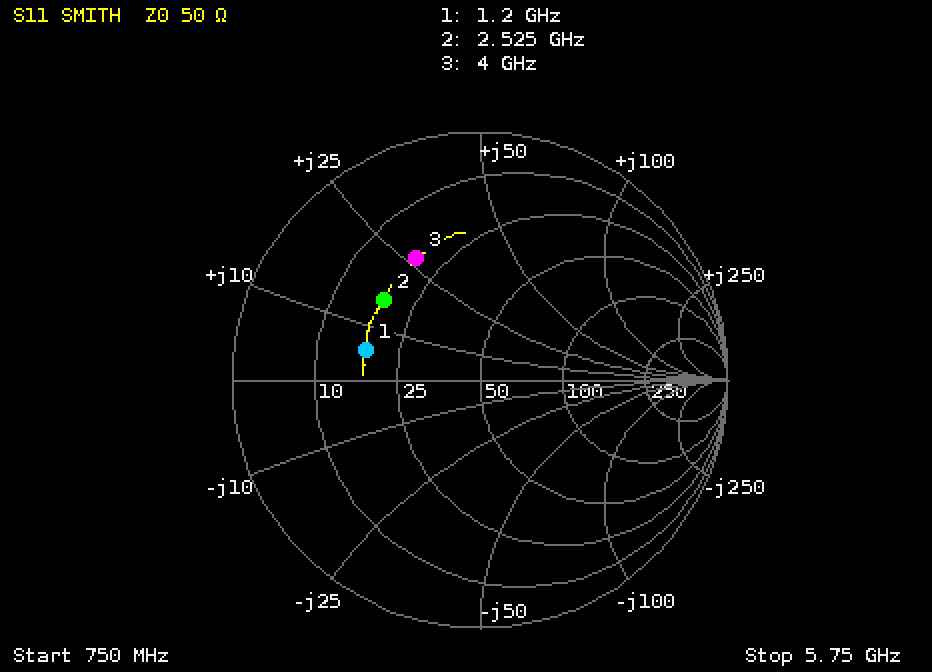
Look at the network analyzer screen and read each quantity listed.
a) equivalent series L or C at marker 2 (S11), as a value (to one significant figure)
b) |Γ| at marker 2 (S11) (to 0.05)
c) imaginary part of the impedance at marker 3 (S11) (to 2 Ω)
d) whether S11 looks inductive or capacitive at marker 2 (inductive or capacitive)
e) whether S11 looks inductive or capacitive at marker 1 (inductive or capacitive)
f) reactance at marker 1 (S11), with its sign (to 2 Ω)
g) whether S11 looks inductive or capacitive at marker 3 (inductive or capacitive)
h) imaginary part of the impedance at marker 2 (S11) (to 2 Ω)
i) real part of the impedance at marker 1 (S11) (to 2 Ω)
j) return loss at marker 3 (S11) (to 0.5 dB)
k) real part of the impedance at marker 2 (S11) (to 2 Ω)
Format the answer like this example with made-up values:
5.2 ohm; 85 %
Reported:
1.0 nH; 0.50; +26 Ω; inductive; inductive; +6 Ω; inductive; +16 Ω; 18 Ω; 5.0 dB; 18 Ω
